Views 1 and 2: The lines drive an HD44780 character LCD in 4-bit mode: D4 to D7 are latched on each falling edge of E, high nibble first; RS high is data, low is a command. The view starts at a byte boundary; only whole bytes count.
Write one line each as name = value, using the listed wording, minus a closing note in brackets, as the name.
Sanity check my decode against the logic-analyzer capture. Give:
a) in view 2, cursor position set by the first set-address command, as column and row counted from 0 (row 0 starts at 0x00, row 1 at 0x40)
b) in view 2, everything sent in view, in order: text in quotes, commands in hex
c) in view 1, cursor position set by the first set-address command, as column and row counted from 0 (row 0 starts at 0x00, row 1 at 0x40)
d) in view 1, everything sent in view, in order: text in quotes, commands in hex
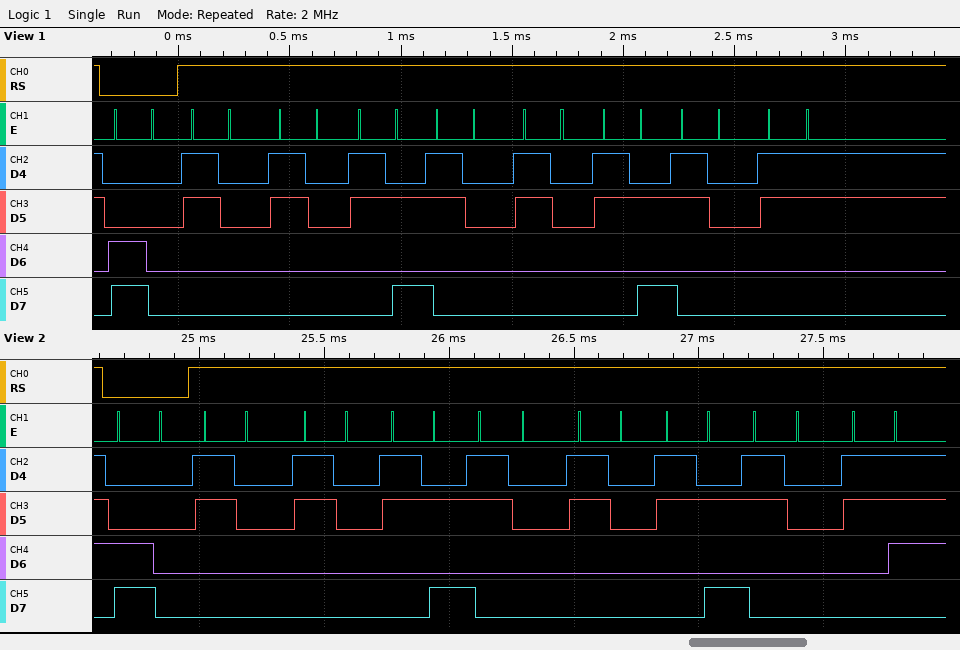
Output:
in view 2, cursor position set by the first set-address command, as column and row counted from 0 = column 0, row 1
in view 2, everything sent in view, in order: text in quotes, commands in hex = 0xC0 "00:00:07"
in view 1, cursor position set by the first set-address command, as column and row counted from 0 = column 0, row 1
in view 1, everything sent in view, in order: text in quotes, commands in hex = 0xC0 "00:00:03"
